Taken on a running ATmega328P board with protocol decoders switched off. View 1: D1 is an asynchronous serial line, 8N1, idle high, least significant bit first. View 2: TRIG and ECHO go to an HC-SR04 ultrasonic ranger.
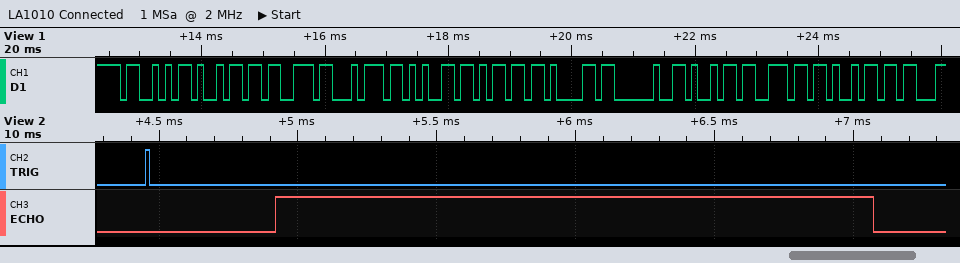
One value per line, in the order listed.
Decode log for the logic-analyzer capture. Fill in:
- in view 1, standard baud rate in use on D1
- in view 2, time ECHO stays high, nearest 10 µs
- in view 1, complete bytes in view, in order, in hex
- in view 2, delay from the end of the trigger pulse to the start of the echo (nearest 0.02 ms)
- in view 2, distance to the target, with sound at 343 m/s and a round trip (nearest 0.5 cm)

9600 baud
2150 µs
0x53 0x69 0x73 0x74 0x65 0x6D 0x61 0x20 0x69 0x6E 0x69
0.46 ms
37 cm
